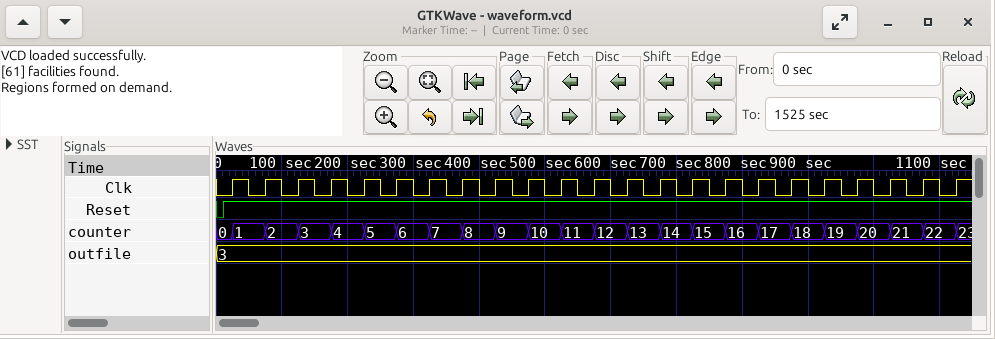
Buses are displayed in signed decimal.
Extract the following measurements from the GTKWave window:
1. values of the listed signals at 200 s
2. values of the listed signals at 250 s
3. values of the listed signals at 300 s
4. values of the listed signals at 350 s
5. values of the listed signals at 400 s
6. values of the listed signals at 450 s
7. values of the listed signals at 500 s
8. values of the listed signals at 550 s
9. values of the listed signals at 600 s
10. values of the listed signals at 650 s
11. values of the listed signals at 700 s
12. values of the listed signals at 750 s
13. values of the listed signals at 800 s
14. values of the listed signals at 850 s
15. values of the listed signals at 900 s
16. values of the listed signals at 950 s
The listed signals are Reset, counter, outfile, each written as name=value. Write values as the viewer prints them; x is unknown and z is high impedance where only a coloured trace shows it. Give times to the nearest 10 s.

Reset=1, counter=4, outfile=3
Reset=1, counter=5, outfile=3
Reset=1, counter=6, outfile=3
Reset=1, counter=7, outfile=3
Reset=1, counter=8, outfile=3
Reset=1, counter=9, outfile=3
Reset=1, counter=10, outfile=3
Reset=1, counter=11, outfile=3
Reset=1, counter=12, outfile=3
Reset=1, counter=13, outfile=3
Reset=1, counter=14, outfile=3
Reset=1, counter=15, outfile=3
Reset=1, counter=16, outfile=3
Reset=1, counter=17, outfile=3
Reset=1, counter=18, outfile=3
Reset=1, counter=19, outfile=3
